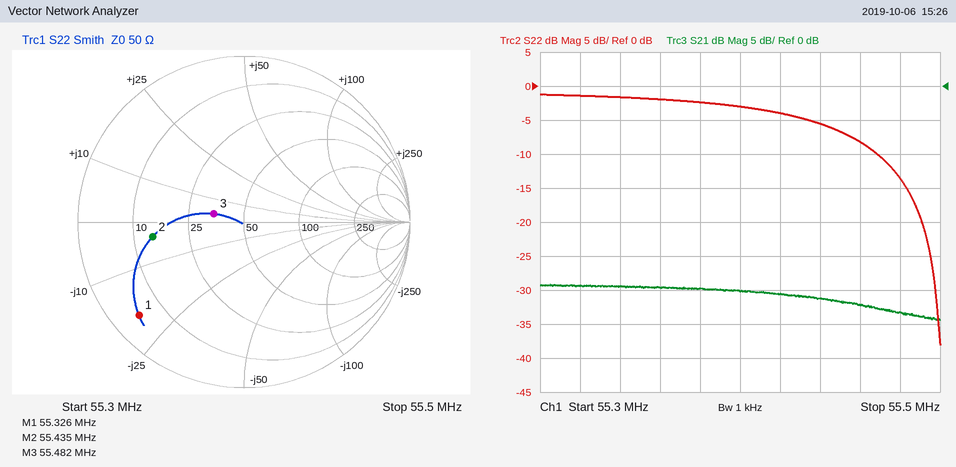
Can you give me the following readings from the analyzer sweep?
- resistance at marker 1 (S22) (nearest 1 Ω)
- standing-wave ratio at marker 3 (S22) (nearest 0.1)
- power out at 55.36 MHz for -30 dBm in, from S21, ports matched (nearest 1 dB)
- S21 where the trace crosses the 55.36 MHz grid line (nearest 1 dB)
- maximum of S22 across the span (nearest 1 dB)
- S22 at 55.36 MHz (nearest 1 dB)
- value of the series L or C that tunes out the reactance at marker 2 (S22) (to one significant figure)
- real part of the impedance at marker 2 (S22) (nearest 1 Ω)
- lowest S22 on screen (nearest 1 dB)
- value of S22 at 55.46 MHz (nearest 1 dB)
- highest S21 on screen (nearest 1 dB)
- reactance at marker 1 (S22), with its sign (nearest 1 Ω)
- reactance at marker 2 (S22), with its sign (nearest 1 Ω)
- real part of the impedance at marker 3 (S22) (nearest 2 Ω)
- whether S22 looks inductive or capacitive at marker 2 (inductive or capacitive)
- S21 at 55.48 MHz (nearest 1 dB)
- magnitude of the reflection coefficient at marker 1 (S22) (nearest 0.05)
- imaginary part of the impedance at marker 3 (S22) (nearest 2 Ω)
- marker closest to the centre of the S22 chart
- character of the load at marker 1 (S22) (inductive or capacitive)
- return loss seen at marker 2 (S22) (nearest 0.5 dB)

5 Ω
1.5
-60 dBm
-30 dB
-1 dB
-2 dB
10 nH
14 Ω
-38 dB
-8 dB
-29 dB
-19 Ω
-4 Ω
34 Ω
capacitive
-33 dB
0.85
+4 Ω
marker 3
capacitive
5.0 dB
